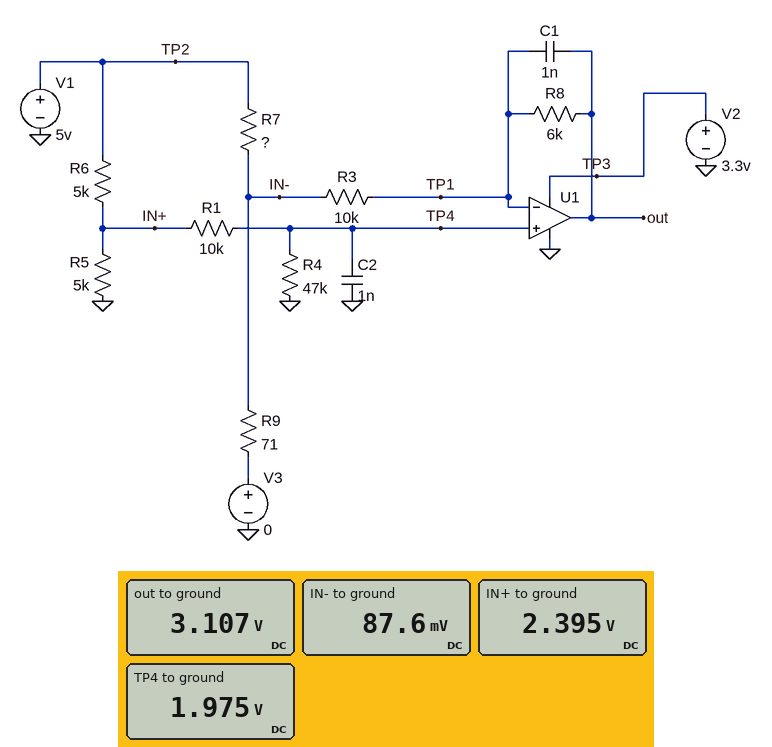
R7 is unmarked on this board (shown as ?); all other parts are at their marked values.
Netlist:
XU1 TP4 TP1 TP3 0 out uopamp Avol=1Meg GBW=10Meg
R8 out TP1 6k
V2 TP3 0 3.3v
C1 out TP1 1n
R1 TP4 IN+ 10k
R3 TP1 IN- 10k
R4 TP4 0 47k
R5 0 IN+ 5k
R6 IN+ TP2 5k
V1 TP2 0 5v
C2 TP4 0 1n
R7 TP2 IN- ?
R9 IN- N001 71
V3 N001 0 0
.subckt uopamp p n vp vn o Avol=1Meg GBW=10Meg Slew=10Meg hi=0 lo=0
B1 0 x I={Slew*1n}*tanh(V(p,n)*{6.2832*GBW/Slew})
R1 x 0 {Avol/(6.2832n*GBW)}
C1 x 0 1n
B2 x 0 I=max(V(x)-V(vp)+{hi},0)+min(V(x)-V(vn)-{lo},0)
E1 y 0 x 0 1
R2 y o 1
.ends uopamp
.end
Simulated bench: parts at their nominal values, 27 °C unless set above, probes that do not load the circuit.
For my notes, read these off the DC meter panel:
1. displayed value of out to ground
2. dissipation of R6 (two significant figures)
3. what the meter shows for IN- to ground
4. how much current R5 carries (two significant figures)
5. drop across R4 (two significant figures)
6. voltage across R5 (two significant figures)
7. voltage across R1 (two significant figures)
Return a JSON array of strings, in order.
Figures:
["3.107 V", "1.4 mW", "87.6 mV", "480 µA", "2.0 V", "2.4 V", "420 mV"]
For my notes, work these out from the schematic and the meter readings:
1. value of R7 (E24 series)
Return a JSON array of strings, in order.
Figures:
["4.7 kΩ"]
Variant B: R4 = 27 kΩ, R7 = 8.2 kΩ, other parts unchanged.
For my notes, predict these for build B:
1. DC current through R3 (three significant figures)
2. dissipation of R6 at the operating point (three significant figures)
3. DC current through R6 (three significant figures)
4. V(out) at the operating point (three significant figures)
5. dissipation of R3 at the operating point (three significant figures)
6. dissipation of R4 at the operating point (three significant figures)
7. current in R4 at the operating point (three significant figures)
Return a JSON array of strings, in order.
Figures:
["165 µA", "1.41 mW", "532 µA", "2.70 V", "274 µW", "108 µW", "63.3 µA"]
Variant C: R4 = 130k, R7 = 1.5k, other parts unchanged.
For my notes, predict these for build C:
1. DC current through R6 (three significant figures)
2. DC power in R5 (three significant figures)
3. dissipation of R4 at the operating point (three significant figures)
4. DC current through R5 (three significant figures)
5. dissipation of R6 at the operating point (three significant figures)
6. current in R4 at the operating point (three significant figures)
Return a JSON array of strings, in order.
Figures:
["509 µA", "1.21 mW", "40.0 µW", "491 µA", "1.29 mW", "17.5 µA"]
